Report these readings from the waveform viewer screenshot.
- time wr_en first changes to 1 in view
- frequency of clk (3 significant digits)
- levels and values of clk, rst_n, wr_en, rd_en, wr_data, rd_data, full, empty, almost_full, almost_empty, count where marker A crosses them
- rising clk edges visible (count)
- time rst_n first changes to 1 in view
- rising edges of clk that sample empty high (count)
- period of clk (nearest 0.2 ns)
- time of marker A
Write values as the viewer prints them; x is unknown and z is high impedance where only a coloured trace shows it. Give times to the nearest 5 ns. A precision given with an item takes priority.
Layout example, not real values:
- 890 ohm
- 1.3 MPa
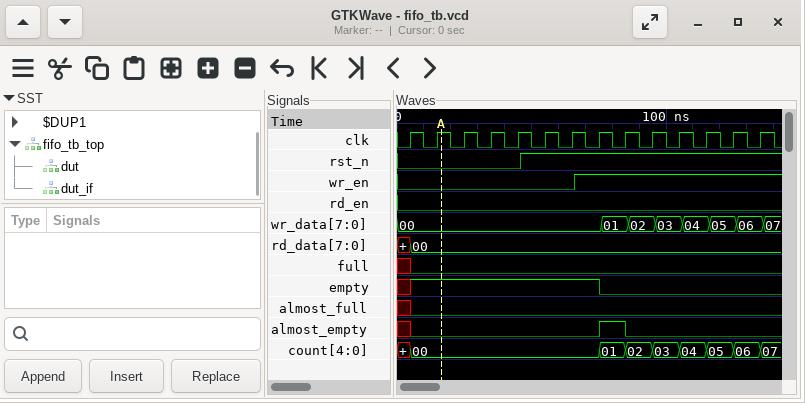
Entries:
- 65 ns
- 100 MHz
- clk=1, rst_n=0, wr_en=0, rd_en=0, wr_data=00, rd_data=00, full=0, empty=1, almost_full=0, almost_empty=0, count=00
- 14
- 45 ns
- 7
- 10 ns
- 15 ns
